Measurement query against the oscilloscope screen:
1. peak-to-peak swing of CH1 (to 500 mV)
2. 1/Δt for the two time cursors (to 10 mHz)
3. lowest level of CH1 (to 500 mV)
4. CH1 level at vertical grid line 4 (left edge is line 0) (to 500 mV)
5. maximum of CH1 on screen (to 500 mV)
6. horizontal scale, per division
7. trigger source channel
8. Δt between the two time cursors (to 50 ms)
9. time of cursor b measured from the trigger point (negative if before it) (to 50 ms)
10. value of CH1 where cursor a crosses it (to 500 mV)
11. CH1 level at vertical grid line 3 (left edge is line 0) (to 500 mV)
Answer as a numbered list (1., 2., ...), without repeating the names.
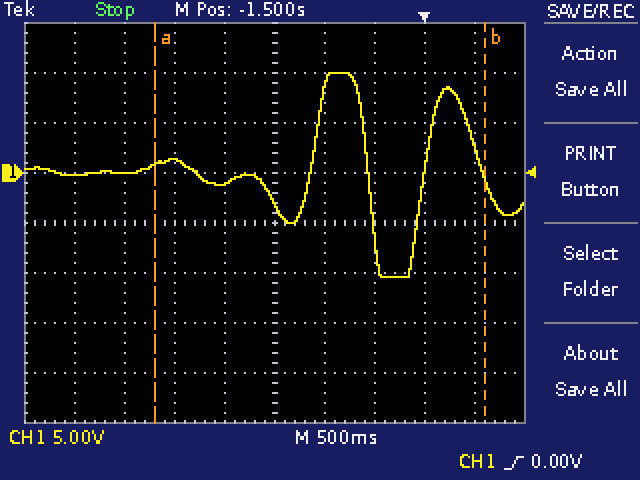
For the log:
1. 20.5 V
2. 300 mHz
3. -10.5 V
4. -1.0 V
5. 10.0 V
6. 500 ms
7. CH1
8. 3.30 s
9. +600 ms
10. 1.0 V
11. 1.5 V
